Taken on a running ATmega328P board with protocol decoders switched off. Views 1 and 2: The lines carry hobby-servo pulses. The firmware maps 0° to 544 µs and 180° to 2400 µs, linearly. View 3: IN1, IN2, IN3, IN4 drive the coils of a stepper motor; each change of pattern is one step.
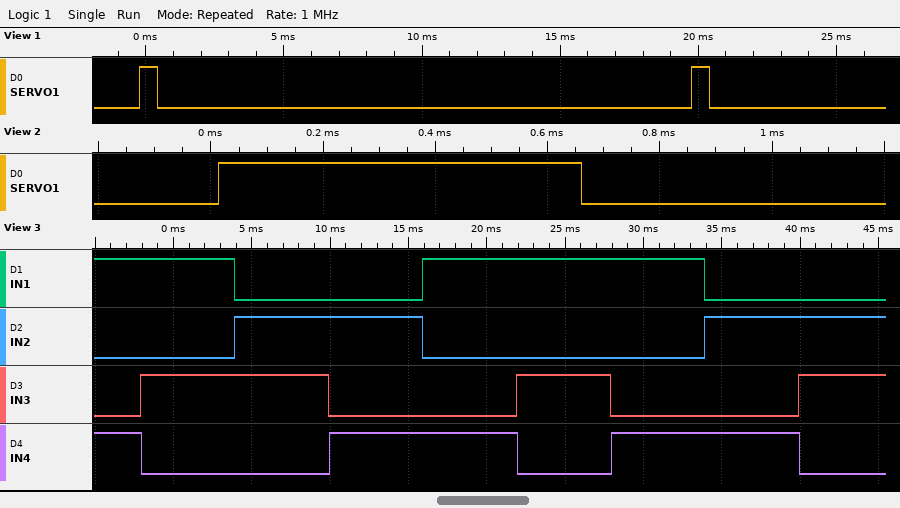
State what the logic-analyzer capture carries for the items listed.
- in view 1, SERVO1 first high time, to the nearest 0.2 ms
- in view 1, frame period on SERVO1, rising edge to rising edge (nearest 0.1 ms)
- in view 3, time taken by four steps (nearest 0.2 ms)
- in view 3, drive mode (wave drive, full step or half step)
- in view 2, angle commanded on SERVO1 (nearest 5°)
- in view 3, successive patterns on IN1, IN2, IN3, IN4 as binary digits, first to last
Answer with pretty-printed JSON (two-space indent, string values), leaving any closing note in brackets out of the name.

{
  "in view 1, SERVO1 first high time, to the nearest 0.2 ms": "0.6 ms",
  "in view 1, frame period on SERVO1, rising edge to rising edge": "20.0 ms",
  "in view 3, time taken by four steps": "24.0 ms",
  "in view 3, drive mode": "full step",
  "in view 2, angle commanded on SERVO1": "10°",
  "in view 3, successive patterns on IN1, IN2, IN3, IN4 as binary digits, first to last": "1001 1010 0110 0101 1001 1010 1001 0101 0110"
}
